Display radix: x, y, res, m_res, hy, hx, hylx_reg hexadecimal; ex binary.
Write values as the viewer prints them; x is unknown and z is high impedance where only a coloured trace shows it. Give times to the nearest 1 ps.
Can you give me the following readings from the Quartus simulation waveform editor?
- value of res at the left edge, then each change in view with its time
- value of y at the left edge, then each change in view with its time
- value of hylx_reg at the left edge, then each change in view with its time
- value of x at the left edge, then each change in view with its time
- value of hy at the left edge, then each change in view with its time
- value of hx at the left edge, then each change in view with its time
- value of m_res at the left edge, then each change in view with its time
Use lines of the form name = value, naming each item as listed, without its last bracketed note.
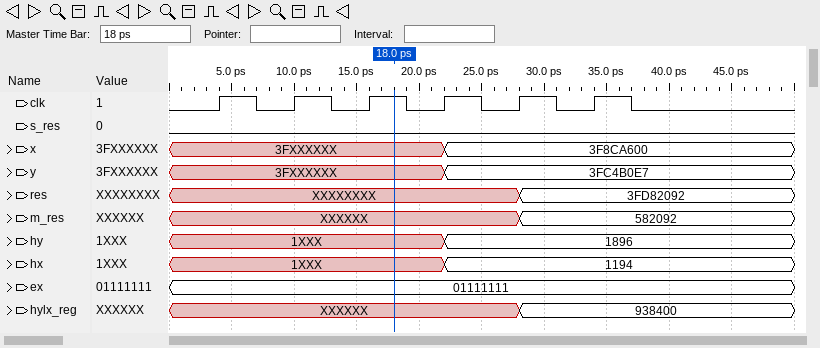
value of res at the left edge, then each change in view with its time = XXXXXXXX, 3FD82092 at 28 ps
value of y at the left edge, then each change in view with its time = 3FXXXXXX, 3FC4B0E7 at 22 ps
value of hylx_reg at the left edge, then each change in view with its time = XXXXXX, 938400 at 28 ps
value of x at the left edge, then each change in view with its time = 3FXXXXXX, 3F8CA600 at 22 ps
value of hy at the left edge, then each change in view with its time = 1XXX, 1896 at 22 ps
value of hx at the left edge, then each change in view with its time = 1XXX, 1194 at 22 ps
value of m_res at the left edge, then each change in view with its time = XXXXXX, 582092 at 28 ps
